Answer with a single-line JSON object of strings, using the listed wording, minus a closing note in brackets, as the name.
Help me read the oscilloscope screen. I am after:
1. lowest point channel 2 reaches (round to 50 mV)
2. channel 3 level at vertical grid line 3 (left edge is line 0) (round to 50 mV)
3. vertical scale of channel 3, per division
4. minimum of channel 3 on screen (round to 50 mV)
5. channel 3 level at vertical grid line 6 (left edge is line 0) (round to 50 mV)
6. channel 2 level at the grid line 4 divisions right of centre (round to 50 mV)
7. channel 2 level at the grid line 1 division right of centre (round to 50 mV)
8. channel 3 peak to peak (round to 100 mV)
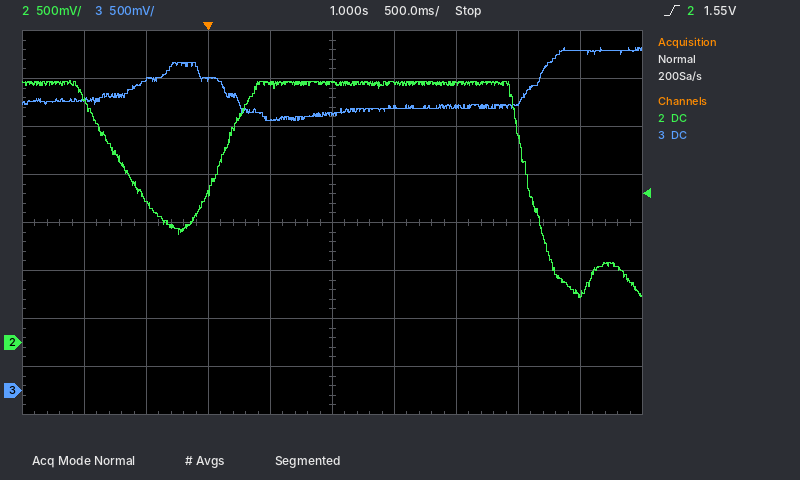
{"lowest point channel 2 reaches": "450 mV", "channel 3 level at vertical grid line 3 (left edge is line 0)": "3.25 V", "vertical scale of channel 3, per division": "500 mV", "minimum of channel 3 on screen": "2.80 V", "channel 3 level at vertical grid line 6 (left edge is line 0)": "2.95 V", "channel 2 level at the grid line 4 divisions right of centre": "500 mV", "channel 2 level at the grid line 1 division right of centre": "2.70 V", "channel 3 peak to peak": "800 mV"}
